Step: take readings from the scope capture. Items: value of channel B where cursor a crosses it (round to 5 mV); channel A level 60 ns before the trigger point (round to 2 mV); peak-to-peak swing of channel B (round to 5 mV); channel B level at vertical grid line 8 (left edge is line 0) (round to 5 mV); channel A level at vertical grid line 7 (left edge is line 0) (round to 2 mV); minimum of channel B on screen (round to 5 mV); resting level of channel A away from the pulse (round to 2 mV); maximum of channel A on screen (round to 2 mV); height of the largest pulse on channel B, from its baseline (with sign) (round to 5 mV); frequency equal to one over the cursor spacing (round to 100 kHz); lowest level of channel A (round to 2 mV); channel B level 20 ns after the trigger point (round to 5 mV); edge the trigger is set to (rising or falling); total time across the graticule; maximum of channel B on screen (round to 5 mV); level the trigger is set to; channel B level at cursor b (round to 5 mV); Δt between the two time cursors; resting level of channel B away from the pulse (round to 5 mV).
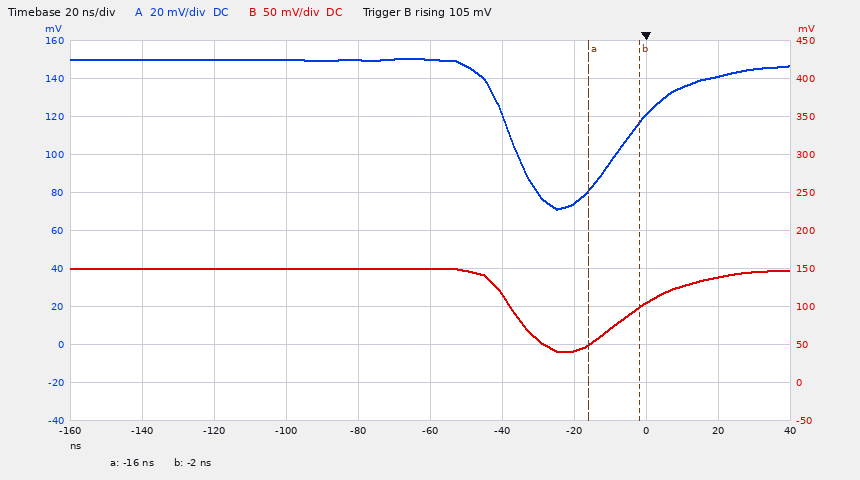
50 mV
150 mV
110 mV
105 mV
74 mV
40 mV
150 mV
150 mV
-110 mV
71.4 MHz
72 mV
140 mV
rising
200 ns
150 mV
105 mV
100 mV
14 ns
150 mV
